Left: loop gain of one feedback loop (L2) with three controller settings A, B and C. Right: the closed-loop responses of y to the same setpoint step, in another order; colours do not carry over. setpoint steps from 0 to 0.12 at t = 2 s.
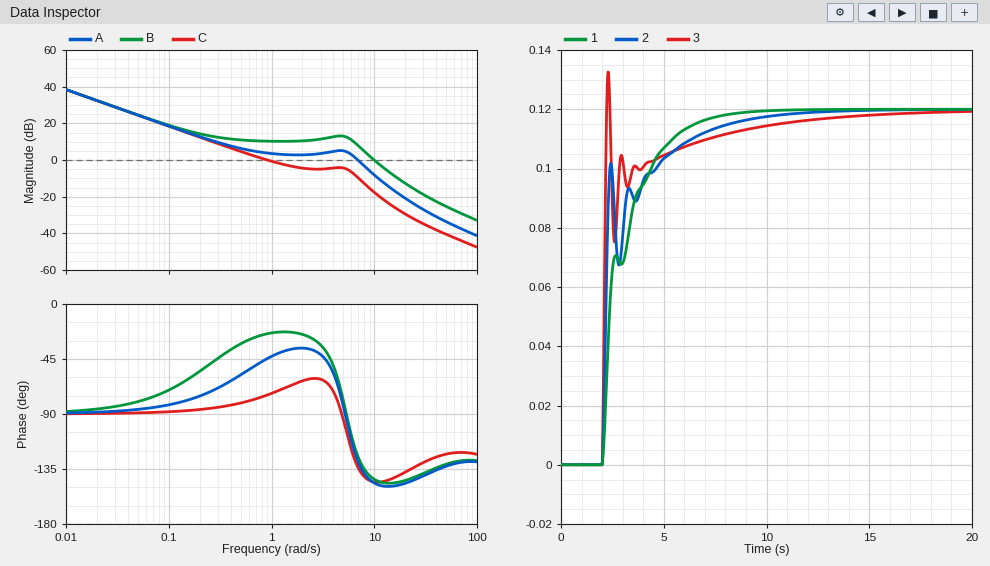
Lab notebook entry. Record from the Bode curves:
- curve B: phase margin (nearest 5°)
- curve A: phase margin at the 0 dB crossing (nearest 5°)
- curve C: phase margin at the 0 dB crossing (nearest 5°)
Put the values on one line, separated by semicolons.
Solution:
35°; 50°; 105°
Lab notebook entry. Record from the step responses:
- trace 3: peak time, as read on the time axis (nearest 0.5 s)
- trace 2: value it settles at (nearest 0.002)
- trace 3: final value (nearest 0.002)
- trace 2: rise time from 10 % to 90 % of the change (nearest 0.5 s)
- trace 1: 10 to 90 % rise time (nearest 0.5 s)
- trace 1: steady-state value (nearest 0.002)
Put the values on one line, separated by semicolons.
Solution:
2.5 s; 0.120; 0.120; 4.0 s; 3.0 s; 0.120
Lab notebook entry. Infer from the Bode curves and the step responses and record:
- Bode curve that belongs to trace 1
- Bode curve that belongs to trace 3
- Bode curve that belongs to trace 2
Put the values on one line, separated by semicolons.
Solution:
C; B; A
